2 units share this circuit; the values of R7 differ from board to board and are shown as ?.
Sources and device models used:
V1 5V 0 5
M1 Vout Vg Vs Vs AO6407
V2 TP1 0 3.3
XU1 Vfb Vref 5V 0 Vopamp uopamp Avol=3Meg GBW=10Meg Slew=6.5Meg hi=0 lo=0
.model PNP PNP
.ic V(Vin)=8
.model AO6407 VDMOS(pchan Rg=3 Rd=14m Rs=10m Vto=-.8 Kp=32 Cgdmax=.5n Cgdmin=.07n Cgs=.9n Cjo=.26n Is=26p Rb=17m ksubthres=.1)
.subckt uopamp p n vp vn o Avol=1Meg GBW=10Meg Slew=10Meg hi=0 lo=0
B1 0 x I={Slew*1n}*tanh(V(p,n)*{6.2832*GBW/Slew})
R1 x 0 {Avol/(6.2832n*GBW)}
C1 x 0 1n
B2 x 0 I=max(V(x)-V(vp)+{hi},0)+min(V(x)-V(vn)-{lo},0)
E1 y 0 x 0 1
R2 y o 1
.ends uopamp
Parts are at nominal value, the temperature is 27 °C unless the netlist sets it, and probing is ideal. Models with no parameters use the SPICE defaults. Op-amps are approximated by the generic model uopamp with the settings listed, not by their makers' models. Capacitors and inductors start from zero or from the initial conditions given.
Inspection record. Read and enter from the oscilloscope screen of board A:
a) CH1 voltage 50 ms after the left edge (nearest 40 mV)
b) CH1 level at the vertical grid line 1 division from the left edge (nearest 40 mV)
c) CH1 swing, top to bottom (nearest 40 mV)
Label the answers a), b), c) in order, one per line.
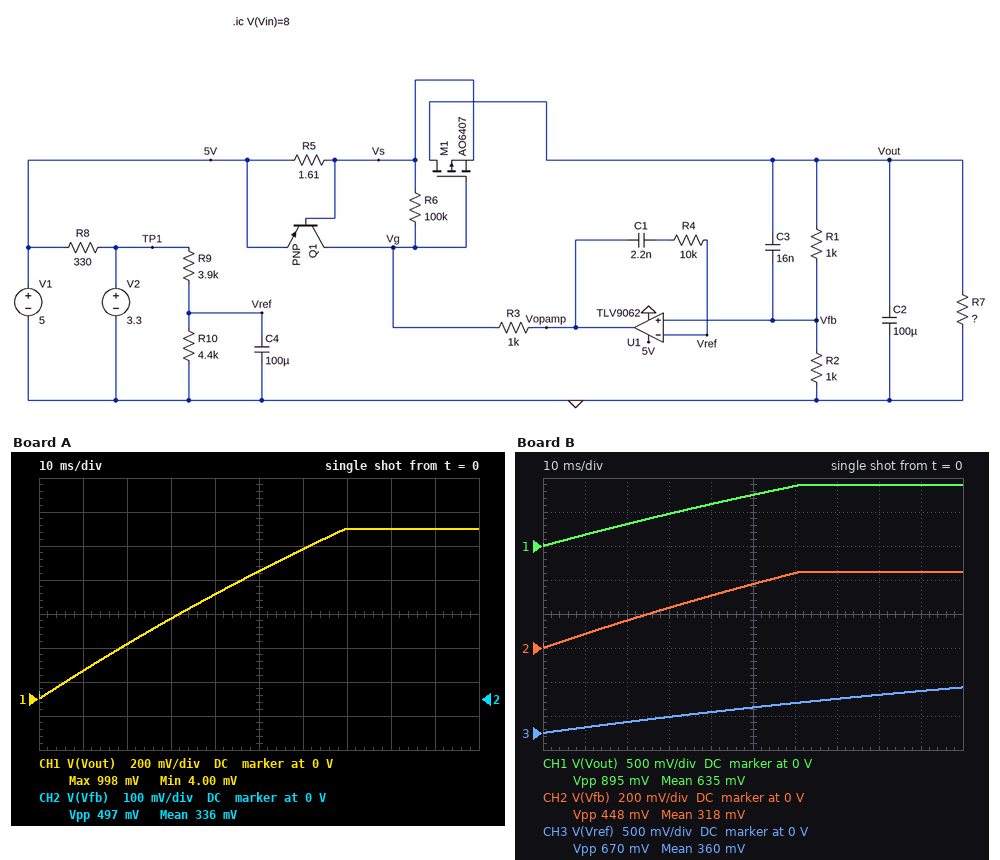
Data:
a) 760 mV
b) 160 mV
c) 1.00 V
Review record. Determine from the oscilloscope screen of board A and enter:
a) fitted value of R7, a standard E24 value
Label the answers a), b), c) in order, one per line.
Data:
a) 2 Ω
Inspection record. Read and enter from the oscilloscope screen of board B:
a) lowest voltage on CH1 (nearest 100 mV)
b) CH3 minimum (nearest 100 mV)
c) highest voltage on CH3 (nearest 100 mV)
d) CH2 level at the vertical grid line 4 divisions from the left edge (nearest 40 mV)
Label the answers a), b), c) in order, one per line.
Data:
a) 0 V
b) 0 V
c) 700 mV
d) 320 mV
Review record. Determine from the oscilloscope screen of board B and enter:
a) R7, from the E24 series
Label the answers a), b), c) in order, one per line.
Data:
a) 1.8 Ω
